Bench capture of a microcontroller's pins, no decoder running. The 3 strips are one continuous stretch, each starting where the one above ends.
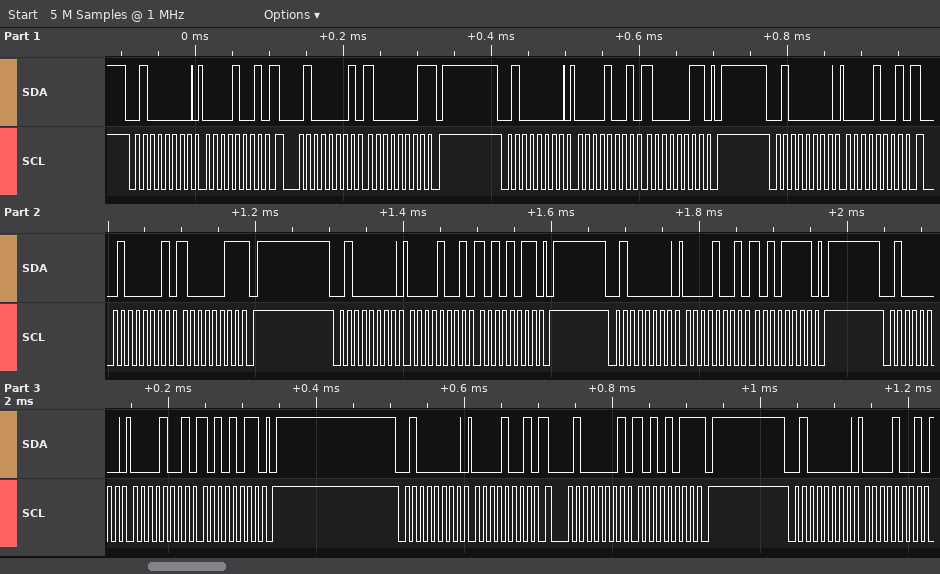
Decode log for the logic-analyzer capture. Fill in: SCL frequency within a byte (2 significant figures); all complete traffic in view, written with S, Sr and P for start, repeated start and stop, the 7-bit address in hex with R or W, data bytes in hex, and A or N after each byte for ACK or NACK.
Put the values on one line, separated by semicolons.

100 kHz; S 20W A 09 A Sr 20R A 81 N P S 20W A 09 A 83 A P S 20W A 09 A Sr 20R A 83 N P S 20W A 09 A AB A P S 20W A 09 A AF A P S 20W A 09 A AB A P S 20W A 09 A Sr 20R A AB N P S 20W A 09 A
